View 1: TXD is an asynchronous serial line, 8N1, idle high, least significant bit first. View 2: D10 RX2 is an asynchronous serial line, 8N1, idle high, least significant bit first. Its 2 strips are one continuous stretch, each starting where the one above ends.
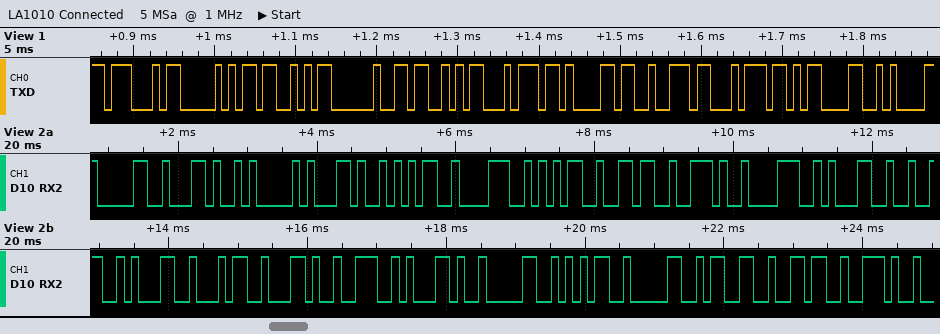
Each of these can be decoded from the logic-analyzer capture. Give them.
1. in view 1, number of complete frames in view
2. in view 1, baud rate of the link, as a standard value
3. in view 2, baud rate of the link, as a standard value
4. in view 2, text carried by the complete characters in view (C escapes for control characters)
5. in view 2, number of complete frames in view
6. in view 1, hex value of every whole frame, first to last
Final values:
11
115200 baud
9600 baud
"0,A,5856.81214,N,05036."
23
47 50 53 20 53 74 61 72 74 0D 0A
